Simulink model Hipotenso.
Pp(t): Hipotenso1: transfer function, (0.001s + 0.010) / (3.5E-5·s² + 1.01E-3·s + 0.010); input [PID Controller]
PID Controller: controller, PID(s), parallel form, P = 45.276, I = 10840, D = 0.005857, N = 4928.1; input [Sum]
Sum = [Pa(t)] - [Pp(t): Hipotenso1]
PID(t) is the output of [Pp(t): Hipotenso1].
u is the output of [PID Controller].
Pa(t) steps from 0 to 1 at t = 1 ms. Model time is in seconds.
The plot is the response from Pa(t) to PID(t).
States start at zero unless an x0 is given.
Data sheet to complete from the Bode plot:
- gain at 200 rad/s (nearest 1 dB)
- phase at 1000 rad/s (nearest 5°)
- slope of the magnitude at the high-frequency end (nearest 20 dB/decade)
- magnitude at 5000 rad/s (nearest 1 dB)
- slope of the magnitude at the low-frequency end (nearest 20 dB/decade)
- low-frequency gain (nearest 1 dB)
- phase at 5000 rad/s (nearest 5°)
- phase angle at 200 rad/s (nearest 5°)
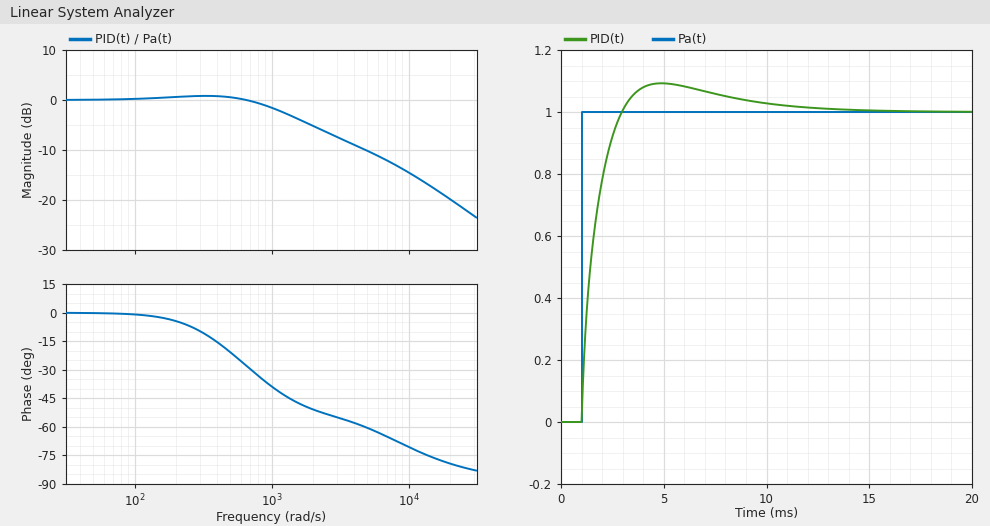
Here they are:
1 dB
-40°
-20 dB/decade
-10 dB
0 dB/decade
0 dB
-60°
-5°
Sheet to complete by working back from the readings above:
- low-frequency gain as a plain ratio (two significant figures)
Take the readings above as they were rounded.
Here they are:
1.0
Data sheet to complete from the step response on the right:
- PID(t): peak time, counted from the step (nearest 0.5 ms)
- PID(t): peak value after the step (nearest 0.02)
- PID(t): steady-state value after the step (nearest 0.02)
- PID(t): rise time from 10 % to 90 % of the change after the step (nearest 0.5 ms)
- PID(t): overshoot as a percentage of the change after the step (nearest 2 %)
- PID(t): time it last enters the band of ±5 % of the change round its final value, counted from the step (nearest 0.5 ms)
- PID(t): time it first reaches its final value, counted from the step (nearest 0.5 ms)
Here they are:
4.0 ms
1.10
1.00
1.5 ms
10 %
7.0 ms
2.0 ms
